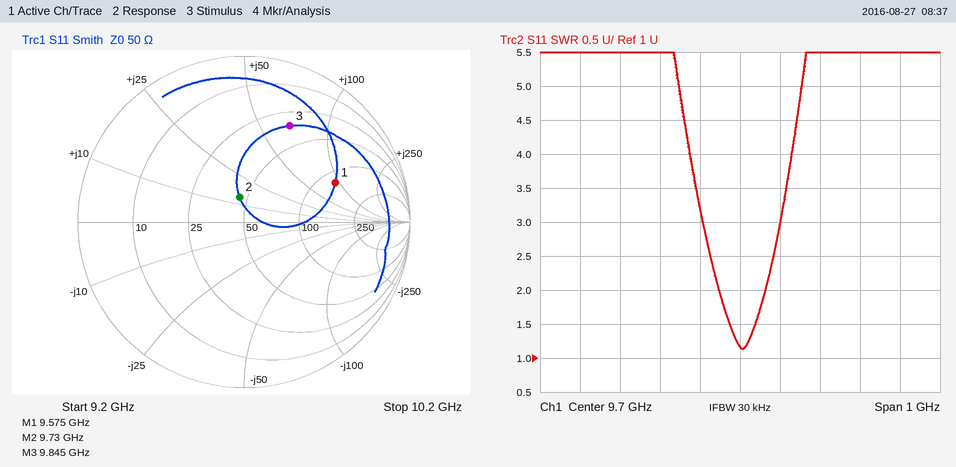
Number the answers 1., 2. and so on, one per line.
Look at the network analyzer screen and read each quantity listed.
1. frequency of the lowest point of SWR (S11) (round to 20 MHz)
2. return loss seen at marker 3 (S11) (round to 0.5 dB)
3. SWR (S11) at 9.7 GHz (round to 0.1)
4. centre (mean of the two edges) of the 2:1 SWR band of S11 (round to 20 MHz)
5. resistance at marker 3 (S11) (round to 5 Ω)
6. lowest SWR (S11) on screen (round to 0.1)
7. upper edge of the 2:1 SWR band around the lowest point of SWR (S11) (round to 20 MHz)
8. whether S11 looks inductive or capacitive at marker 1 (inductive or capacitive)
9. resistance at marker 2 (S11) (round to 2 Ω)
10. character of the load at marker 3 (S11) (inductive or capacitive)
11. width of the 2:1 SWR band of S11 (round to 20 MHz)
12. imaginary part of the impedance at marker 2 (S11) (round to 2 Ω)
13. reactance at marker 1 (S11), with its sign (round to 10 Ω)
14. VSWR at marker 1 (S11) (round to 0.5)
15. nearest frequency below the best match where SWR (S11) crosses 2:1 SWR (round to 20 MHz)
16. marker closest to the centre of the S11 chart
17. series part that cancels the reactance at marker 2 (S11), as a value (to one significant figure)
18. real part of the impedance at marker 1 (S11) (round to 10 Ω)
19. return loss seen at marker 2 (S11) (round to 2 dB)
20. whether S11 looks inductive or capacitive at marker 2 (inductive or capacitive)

1. 9.70 GHz
2. 4.0 dB
3. 1.2
4. 9.70 GHz
5. 35 Ω
6. 1.1
7. 9.76 GHz
8. inductive
9. 46 Ω
10. inductive
11. 120 MHz
12. +14 Ω
13. +90 Ω
14. 4.0
15. 9.64 GHz
16. marker 2
17. 1 pF
18. 120 Ω
19. 16 dB
20. inductive
